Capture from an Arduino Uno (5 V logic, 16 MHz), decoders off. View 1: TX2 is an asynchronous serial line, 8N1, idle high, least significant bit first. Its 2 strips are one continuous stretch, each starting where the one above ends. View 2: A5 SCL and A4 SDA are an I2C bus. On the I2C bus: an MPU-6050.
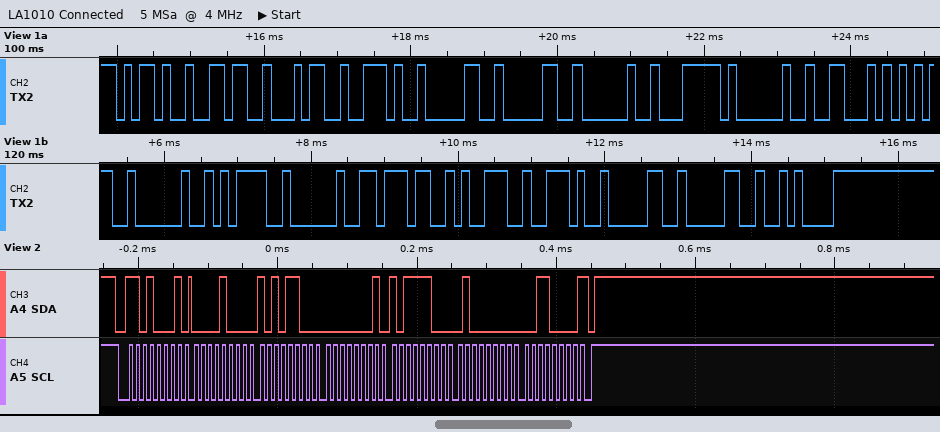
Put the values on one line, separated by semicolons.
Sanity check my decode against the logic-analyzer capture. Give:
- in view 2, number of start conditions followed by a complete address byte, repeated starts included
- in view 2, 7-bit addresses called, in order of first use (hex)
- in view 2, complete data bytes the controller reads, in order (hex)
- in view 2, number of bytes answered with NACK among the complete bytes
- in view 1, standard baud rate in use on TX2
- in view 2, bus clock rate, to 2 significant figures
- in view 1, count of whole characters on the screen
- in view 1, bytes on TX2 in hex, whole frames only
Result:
1; 0x68; 08 AC 01 BC 40 30; 1; 9600 baud; 100 kHz; 20; 2D 36 34 2E 30 30 20 7C 20 46 35 20 3D 20 37 39 2E 30 30 0A
